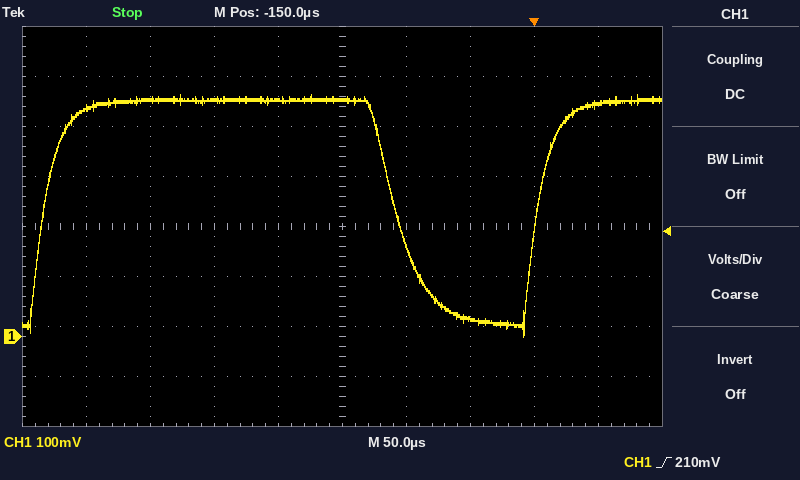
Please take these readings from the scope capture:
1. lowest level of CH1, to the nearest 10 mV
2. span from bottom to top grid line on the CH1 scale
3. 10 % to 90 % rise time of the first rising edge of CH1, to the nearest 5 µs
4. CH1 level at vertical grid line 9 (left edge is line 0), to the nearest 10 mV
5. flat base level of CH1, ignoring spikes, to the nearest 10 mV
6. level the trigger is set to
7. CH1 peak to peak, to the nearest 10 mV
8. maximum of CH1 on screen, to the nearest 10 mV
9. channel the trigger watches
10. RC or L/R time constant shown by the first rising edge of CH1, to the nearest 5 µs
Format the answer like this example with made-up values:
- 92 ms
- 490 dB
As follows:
- 0 mV
- 800 mV
- 30 µs
- 470 mV
- 30 mV
- 210 mV
- 480 mV
- 480 mV
- CH1
- 15 µs
